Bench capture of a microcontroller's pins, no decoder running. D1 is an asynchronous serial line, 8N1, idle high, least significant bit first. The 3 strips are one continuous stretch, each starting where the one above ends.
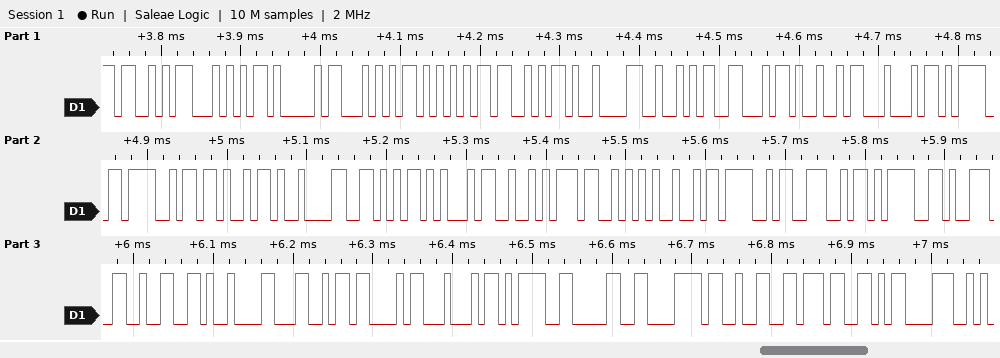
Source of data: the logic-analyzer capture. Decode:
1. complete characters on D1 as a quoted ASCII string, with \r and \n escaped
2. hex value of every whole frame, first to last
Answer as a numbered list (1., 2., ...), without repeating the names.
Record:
1. "STATUS\tRFID=OK\tVERSION=92\tLCD=0x27\r"
2. 53 54 41 54 55 53 09 52 46 49 44 3D 4F 4B 09 56 45 52 53 49 4F 4E 3D 39 32 09 4C 43 44 3D 30 78 32 37 0D
